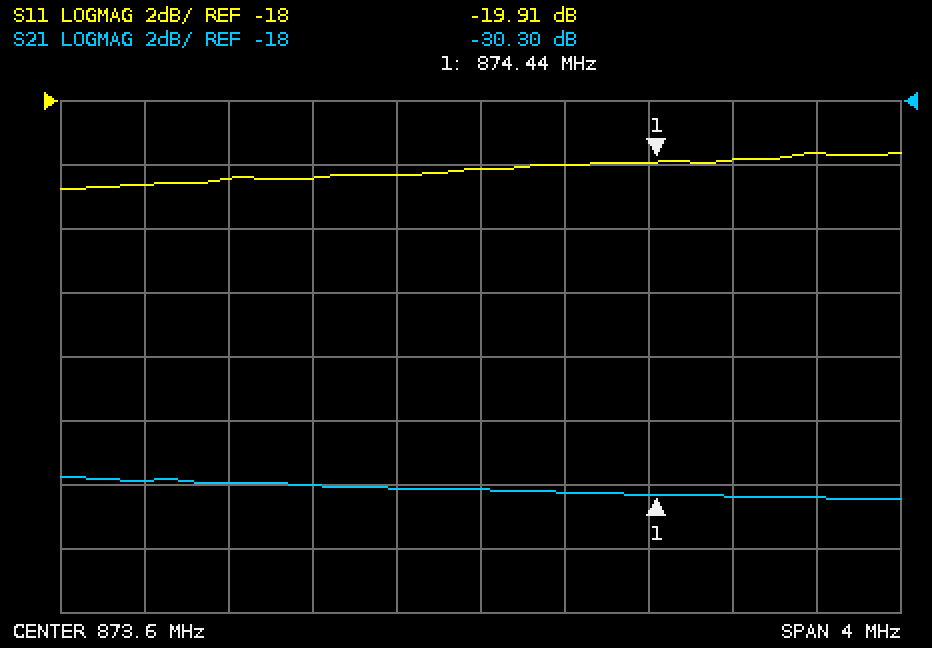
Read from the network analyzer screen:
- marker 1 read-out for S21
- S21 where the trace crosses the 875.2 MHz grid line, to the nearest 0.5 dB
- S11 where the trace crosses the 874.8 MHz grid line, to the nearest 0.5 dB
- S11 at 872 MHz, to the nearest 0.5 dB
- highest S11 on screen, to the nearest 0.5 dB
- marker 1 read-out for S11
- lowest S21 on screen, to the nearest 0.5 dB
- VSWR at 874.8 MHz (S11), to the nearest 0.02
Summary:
-30.30 dB
-30.5 dB
-20.0 dB
-20.5 dB
-19.5 dB
-19.91 dB
-30.5 dB
1.22
